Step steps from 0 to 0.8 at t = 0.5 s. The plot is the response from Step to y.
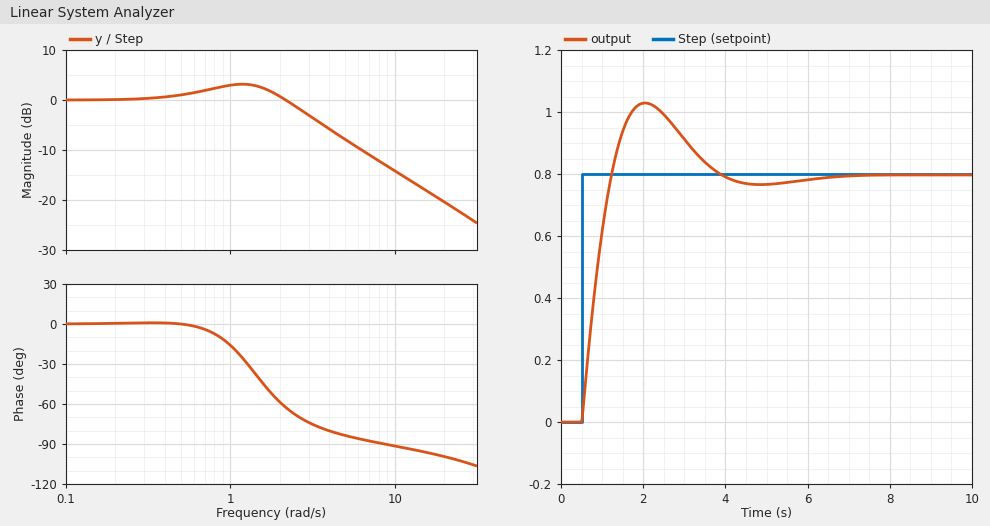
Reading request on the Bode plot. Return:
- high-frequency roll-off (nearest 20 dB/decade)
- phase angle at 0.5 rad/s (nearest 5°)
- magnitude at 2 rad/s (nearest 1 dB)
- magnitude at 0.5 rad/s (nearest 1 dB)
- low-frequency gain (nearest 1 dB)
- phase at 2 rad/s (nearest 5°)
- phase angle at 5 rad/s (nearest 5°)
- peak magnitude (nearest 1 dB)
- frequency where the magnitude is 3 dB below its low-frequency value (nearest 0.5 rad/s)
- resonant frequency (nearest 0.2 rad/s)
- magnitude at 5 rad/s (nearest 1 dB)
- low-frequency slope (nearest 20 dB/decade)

-20 dB/decade
0°
1 dB
1 dB
0 dB
-60°
-85°
3 dB
3.0 rad/s
1.2 rad/s
-8 dB
0 dB/decade
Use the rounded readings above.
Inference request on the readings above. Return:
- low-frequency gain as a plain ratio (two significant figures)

1.0
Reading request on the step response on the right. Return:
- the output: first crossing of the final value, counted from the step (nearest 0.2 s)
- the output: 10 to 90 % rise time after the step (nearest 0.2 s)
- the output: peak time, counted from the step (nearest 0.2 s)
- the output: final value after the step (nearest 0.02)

0.8 s
0.6 s
1.6 s
0.80
